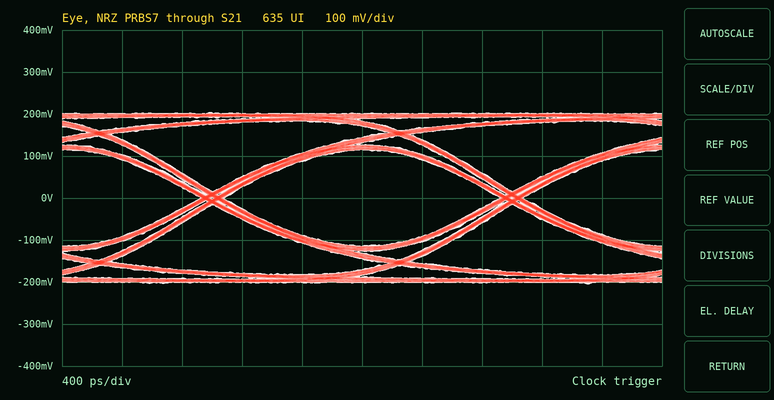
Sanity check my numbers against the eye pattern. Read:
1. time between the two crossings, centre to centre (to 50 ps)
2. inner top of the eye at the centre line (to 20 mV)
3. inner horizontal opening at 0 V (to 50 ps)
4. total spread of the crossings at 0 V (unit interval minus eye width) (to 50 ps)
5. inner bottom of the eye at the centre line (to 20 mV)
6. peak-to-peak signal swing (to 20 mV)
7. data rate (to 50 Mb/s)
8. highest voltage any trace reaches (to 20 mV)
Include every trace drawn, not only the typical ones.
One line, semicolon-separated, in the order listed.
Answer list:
2.00 ns; 120 mV; 1.85 ns; 150 ps; -120 mV; 400 mV; 500 Mb/s; 200 mV
